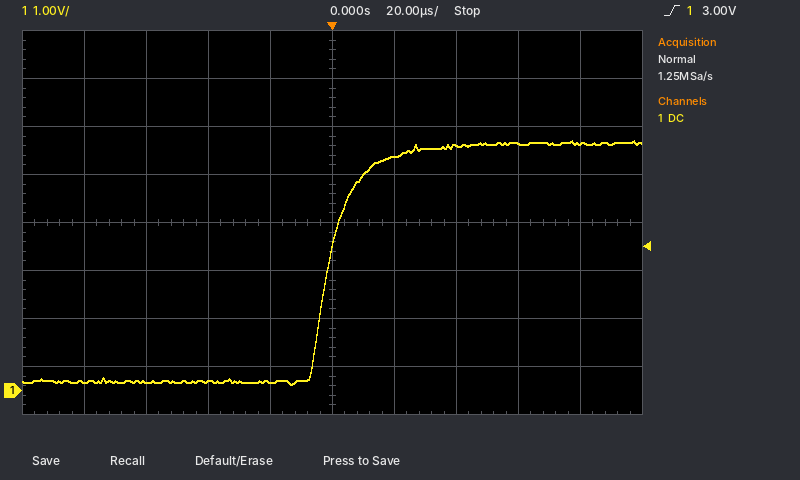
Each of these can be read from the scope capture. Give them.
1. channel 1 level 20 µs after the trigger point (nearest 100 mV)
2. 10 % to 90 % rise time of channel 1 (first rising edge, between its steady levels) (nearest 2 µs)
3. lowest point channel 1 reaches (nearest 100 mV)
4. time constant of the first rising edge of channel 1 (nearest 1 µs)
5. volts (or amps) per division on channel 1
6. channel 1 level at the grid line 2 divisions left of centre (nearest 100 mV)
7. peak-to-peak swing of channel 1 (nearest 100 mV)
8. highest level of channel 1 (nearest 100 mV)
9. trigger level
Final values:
4.9 V
18 µs
100 mV
8 µs
1 V
200 mV
5.1 V
5.2 V
3.00 V
